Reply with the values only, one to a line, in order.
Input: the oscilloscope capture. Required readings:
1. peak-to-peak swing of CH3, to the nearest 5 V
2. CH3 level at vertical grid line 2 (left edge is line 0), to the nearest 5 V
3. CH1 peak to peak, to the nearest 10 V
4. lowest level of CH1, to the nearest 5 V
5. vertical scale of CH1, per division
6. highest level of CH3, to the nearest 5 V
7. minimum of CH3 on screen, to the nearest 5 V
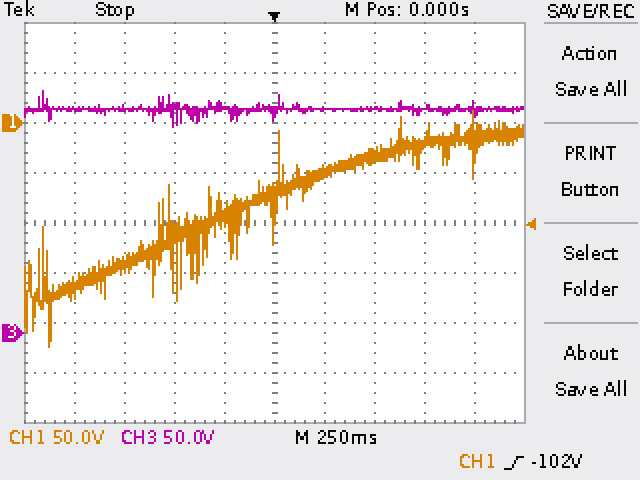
35 V
225 V
240 V
-225 V
50 V
240 V
205 V
